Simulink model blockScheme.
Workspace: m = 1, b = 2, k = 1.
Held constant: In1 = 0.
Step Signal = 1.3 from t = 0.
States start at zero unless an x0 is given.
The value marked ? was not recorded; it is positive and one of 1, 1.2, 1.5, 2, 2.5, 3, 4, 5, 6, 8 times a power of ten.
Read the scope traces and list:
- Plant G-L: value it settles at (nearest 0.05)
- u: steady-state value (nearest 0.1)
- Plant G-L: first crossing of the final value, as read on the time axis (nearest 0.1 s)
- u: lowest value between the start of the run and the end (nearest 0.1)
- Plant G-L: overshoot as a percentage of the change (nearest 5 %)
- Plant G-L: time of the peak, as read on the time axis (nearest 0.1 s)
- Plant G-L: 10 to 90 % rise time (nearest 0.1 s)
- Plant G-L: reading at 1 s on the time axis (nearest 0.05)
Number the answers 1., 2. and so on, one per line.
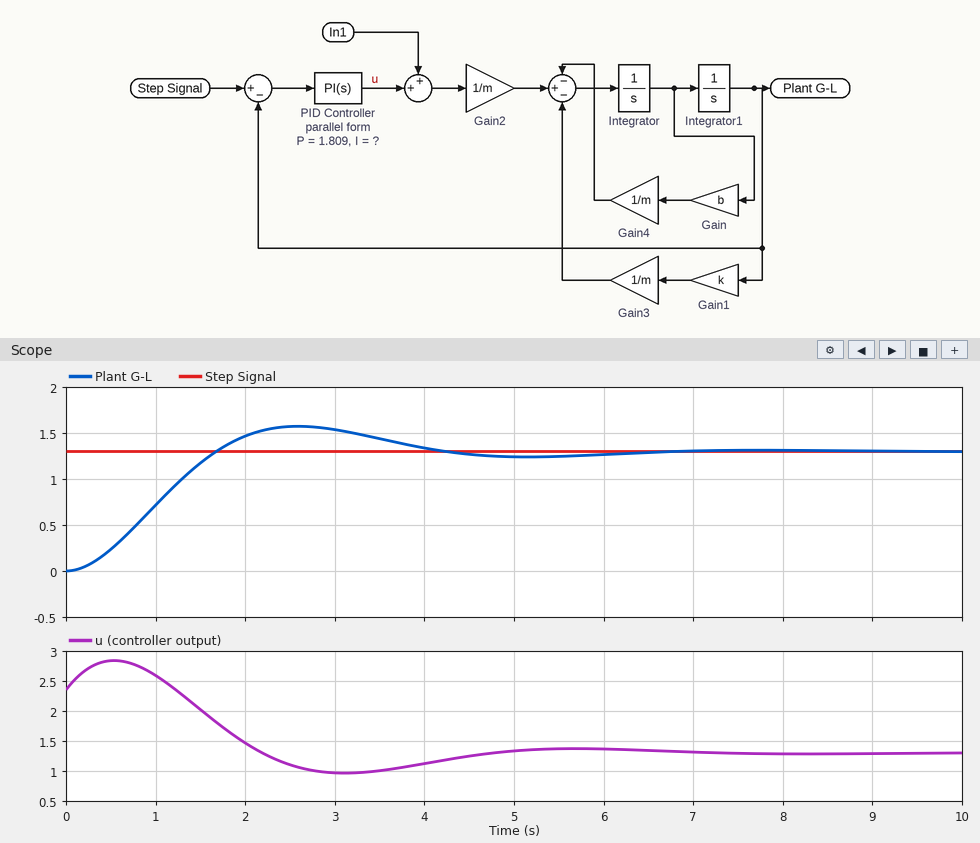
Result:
1. 1.30
2. 1.3
3. 1.7 s
4. 1.0
5. 20 %
6. 2.6 s
7. 1.1 s
8. 0.70
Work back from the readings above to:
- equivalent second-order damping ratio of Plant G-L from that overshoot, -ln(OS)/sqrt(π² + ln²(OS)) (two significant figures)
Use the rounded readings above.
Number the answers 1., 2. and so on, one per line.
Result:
1. 0.46
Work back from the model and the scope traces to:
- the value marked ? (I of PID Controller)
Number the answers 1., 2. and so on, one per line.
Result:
1. 1.5
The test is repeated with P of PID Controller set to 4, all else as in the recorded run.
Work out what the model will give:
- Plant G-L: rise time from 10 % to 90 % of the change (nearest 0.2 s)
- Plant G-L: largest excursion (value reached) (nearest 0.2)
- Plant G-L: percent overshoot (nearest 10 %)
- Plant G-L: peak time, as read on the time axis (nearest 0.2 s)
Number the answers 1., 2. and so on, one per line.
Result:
1. 0.8 s
2. 1.6
3. 20 %
4. 1.6 s
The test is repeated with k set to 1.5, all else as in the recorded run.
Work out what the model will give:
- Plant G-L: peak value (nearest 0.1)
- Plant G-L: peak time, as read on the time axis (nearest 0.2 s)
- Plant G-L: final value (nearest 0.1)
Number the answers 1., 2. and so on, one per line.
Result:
1. 1.4
2. 2.4 s
3. 1.3
